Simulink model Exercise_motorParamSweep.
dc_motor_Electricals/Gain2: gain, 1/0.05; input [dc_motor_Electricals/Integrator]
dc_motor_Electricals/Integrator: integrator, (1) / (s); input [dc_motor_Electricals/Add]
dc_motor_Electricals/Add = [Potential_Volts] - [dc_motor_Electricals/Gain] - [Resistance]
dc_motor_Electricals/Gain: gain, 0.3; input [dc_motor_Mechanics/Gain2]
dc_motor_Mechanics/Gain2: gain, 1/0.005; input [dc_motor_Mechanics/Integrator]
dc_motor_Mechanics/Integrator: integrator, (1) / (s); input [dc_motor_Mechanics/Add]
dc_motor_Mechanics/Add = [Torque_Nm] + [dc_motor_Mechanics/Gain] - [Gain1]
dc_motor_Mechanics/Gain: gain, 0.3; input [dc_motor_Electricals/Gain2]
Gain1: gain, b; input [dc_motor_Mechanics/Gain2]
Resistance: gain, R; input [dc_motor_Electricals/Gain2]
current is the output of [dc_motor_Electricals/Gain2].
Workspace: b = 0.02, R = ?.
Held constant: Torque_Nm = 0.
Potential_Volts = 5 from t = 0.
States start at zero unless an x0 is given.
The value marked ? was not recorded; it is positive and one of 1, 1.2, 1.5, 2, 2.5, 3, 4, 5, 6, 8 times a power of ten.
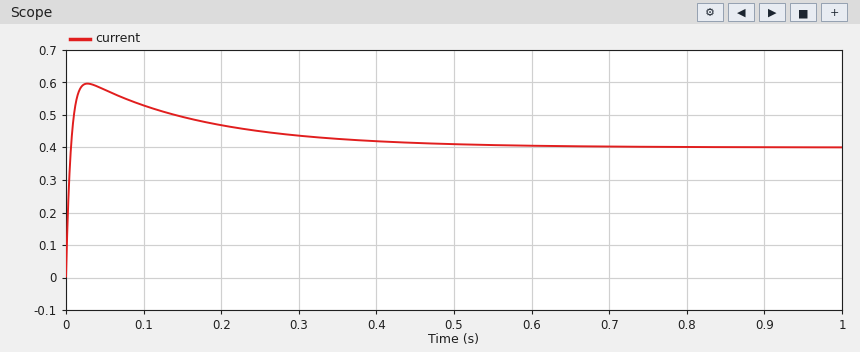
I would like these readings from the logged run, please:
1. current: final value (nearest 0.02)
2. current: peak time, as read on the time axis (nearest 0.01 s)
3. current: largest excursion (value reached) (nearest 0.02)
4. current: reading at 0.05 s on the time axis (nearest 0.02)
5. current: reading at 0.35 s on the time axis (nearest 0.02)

0.40
0.03 s
0.60
0.58
0.42
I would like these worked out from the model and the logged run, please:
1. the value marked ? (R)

8
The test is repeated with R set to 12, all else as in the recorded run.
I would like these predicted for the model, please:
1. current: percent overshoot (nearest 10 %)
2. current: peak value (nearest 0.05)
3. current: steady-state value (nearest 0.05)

30 %
0.40
0.30
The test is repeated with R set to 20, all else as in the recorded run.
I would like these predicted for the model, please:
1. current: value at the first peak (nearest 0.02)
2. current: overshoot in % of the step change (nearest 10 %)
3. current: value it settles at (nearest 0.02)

0.24
20 %
0.20
